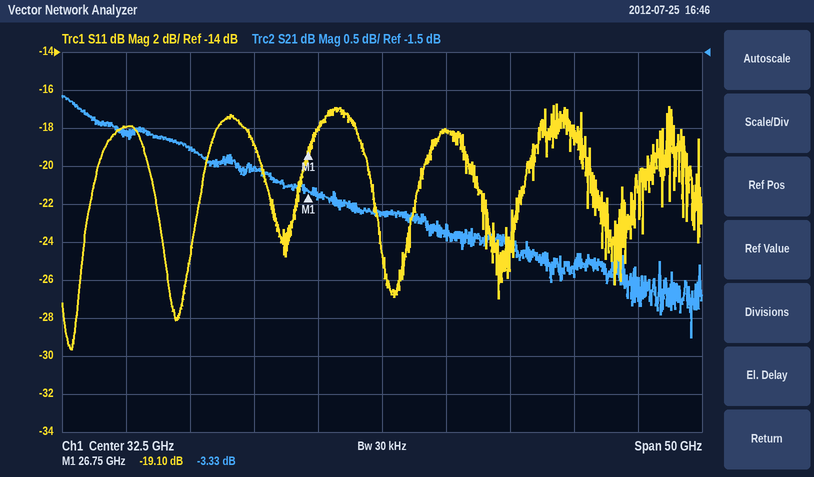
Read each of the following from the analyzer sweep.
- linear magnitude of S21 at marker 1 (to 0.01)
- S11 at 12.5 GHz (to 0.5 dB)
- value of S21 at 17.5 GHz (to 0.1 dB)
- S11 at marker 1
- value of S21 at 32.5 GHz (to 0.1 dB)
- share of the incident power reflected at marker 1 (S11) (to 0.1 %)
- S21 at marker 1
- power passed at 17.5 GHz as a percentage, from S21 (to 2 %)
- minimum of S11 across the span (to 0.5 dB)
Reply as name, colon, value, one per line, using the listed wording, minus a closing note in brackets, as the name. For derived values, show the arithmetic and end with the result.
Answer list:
linear magnitude of S21 at marker 1: 10^(-3.33/20) ≈ 0.68
S11 at 12.5 GHz: -18.0 dB
value of S21 at 17.5 GHz: -2.8 dB
S11 at marker 1: -19.10 dB
value of S21 at 32.5 GHz: -3.6 dB
share of the incident power reflected at marker 1 (S11): 10^(-19.1/10) ≈ 1.2 %
S21 at marker 1: -3.33 dB
power passed at 17.5 GHz as a percentage, from S21: 10^(-2.8/10) ≈ 52 %
minimum of S11 across the span: -29.5 dB
